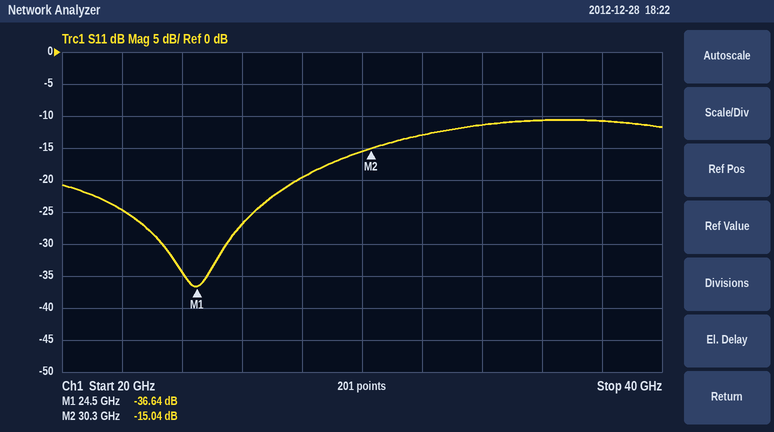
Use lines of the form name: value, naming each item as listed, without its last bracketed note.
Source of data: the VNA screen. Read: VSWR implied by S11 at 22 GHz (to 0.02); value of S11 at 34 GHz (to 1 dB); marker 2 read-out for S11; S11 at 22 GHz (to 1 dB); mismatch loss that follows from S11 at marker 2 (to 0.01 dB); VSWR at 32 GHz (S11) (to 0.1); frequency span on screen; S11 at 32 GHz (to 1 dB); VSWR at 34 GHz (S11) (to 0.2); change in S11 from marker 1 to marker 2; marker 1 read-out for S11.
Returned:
VSWR implied by S11 at 22 GHz: 1.12
value of S11 at 34 GHz: -11 dB
marker 2 read-out for S11: -15.04 dB
S11 at 22 GHz: -25 dB
mismatch loss that follows from S11 at marker 2: 0.14 dB
VSWR at 32 GHz (S11): 1.6
frequency span on screen: 20 GHz
S11 at 32 GHz: -13 dB
VSWR at 34 GHz (S11): 1.8
change in S11 from marker 1 to marker 2: 21.60 dB
marker 1 read-out for S11: -36.64 dB
